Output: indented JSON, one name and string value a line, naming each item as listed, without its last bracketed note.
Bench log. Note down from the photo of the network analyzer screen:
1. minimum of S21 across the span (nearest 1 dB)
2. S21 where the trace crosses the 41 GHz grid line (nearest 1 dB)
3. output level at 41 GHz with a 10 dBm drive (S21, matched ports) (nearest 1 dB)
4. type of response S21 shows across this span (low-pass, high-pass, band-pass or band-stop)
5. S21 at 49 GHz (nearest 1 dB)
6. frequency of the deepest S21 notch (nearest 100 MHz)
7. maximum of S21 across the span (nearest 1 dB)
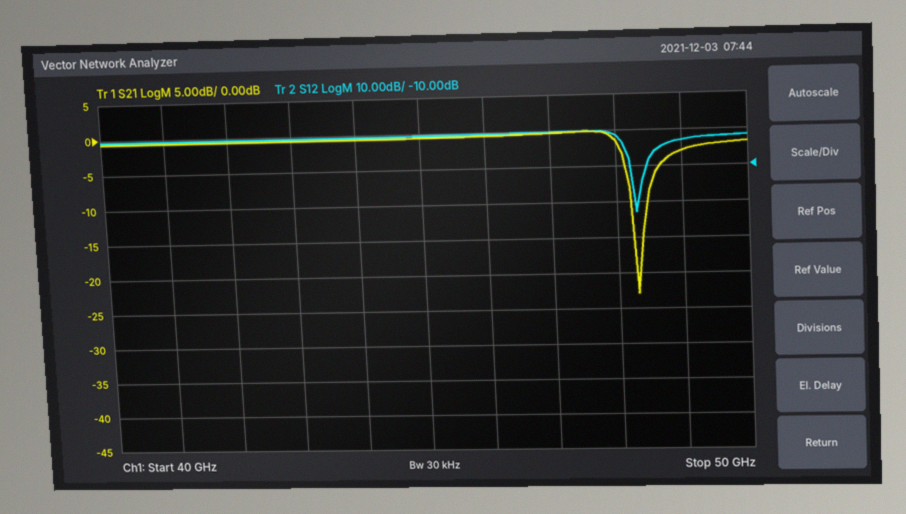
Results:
{
  "minimum of S21 across the span": "-23 dB",
  "S21 where the trace crosses the 41 GHz grid line": "-1 dB",
  "output level at 41 GHz with a 10 dBm drive (S21, matched ports)": "9 dBm",
  "type of response S21 shows across this span": "band-stop",
  "S21 at 49 GHz": "-3 dB",
  "frequency of the deepest S21 notch": "48.3 GHz",
  "maximum of S21 across the span": "0 dB"
}
